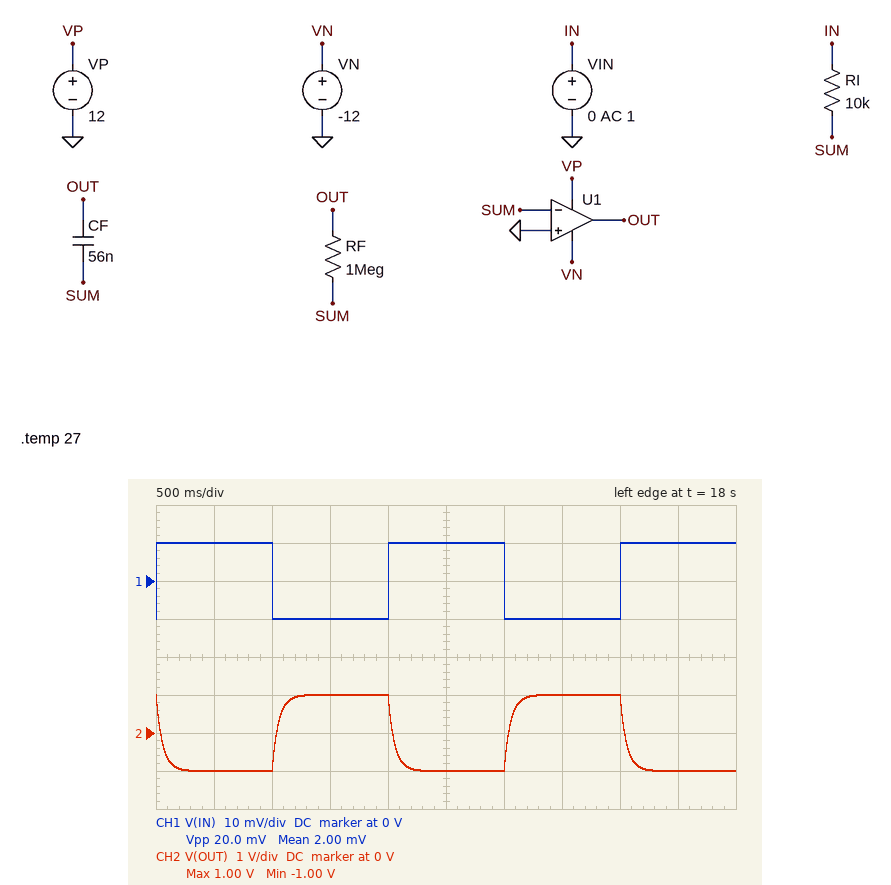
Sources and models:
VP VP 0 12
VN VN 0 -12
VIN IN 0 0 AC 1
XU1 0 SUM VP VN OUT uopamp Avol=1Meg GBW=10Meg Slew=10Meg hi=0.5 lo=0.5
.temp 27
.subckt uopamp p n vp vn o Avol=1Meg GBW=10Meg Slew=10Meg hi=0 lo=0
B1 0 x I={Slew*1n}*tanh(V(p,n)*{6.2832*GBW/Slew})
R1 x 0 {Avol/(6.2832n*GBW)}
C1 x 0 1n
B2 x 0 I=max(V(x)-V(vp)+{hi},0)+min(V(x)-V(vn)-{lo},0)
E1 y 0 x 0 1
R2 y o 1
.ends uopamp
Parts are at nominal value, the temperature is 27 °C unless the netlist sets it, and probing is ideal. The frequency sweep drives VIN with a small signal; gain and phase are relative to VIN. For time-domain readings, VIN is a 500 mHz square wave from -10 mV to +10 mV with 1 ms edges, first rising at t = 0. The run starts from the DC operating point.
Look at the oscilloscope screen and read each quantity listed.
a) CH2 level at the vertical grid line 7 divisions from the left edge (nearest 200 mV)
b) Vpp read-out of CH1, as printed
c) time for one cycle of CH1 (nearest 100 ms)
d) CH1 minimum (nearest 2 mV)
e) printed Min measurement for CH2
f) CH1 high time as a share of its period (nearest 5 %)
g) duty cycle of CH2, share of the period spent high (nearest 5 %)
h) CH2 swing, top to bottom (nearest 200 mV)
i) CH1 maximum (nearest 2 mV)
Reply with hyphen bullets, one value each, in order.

- 1.0 V
- 20.0 mV
- 2.0 s
- -10 mV
- -1.00 V
- 50 %
- 50 %
- 2.0 V
- 10 mV
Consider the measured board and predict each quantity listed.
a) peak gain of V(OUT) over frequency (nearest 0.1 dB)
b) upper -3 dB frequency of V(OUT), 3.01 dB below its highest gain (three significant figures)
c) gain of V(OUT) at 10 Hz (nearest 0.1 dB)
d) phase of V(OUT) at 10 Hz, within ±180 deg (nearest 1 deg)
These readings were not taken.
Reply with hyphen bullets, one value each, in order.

- 40.0 dB
- 2.84 Hz
- 28.7 dB
- 106 deg
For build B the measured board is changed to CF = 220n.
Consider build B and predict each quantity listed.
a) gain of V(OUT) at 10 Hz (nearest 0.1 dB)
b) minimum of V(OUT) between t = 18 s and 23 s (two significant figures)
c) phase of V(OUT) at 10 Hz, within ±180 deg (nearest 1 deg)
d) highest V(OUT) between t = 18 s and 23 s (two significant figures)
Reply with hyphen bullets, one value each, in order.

- 17.2 dB
- -980 mV
- 94 deg
- 980 mV
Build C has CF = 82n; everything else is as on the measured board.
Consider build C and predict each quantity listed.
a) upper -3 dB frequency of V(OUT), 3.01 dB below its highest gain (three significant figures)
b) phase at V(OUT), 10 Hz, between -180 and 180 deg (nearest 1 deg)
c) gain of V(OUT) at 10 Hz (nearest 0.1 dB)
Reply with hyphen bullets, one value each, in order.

- 1.94 Hz
- 101 deg
- 25.6 dB
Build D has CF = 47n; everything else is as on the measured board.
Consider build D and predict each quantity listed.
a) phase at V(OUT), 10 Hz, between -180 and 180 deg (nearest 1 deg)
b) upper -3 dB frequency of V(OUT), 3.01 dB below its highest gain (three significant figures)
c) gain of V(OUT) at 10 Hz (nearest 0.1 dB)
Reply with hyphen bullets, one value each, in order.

- 109 deg
- 3.39 Hz
- 30.1 dB
